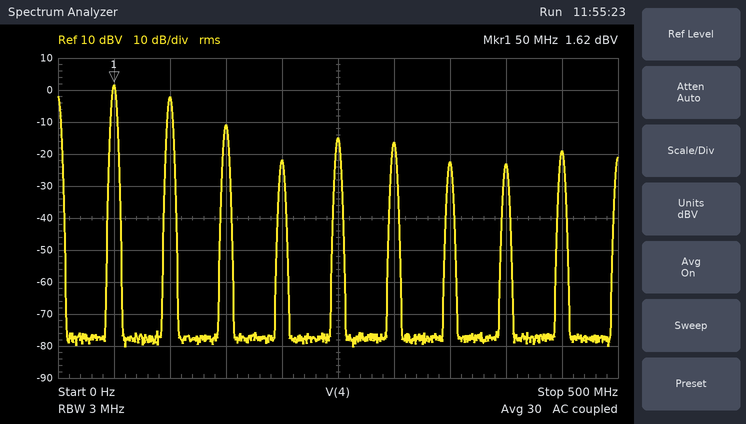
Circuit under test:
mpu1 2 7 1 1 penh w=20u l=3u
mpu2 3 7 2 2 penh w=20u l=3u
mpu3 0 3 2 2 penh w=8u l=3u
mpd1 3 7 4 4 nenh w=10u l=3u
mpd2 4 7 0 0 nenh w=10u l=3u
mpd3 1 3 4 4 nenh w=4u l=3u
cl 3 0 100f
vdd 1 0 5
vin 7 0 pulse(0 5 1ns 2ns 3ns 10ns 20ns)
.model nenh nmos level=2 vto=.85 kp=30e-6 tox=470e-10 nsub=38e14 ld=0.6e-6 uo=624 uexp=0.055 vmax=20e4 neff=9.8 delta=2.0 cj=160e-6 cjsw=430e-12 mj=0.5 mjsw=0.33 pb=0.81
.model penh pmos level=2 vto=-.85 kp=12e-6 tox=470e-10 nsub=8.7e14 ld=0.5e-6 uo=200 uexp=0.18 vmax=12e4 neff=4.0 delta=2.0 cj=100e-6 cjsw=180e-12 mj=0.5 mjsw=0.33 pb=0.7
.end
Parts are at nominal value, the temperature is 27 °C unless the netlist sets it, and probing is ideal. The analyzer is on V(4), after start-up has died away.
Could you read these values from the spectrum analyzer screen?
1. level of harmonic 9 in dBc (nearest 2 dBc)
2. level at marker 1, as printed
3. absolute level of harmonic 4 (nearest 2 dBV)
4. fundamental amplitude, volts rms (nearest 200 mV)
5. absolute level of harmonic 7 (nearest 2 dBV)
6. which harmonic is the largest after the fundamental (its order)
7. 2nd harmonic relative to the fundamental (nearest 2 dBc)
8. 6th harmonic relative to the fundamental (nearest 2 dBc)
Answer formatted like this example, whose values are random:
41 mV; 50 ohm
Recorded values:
-20 dBc; 1.62 dBV; -22 dBV; 1.2 V; -22 dBV; 2; -4 dBc; -18 dBc
